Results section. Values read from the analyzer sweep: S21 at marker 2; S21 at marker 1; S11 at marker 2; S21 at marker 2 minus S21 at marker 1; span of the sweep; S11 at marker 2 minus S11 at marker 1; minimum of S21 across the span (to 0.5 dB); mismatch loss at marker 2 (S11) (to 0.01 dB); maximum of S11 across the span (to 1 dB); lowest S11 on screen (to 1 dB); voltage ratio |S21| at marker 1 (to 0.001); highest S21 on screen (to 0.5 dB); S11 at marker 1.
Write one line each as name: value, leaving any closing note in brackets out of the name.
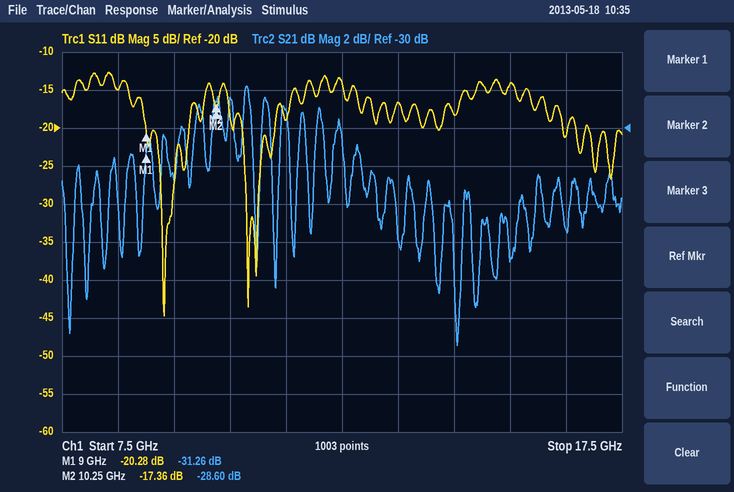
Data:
S21 at marker 2: -28.60 dB
S21 at marker 1: -31.26 dB
S11 at marker 2: -17.36 dB
S21 at marker 2 minus S21 at marker 1: 2.66 dB
span of the sweep: 10 GHz
S11 at marker 2 minus S11 at marker 1: 2.92 dB
minimum of S21 across the span: -41.5 dB
mismatch loss at marker 2 (S11): 0.08 dB
maximum of S11 across the span: -13 dB
lowest S11 on screen: -45 dB
voltage ratio |S21| at marker 1: 0.027
highest S21 on screen: -28.0 dB
S11 at marker 1: -20.28 dB
